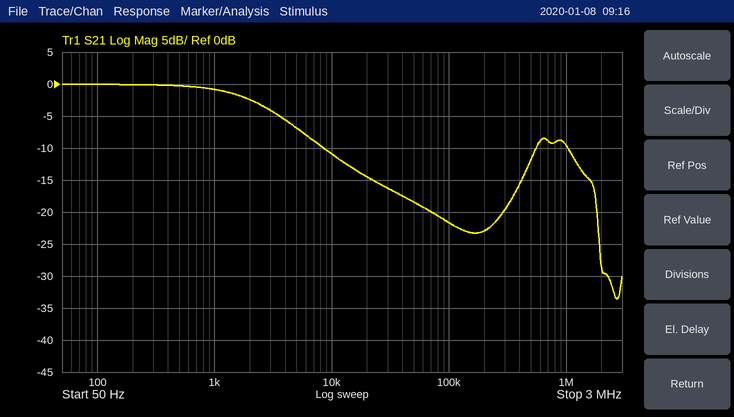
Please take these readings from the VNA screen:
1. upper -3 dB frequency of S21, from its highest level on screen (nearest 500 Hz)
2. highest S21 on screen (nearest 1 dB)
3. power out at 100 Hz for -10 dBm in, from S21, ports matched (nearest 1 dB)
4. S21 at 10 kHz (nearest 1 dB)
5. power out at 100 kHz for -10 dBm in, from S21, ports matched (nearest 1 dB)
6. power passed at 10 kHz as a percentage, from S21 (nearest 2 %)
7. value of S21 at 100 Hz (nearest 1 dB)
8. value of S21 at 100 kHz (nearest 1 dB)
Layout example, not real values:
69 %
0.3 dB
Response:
2.5 kHz
0 dB
-10 dBm
-11 dB
-32 dBm
8 %
0 dB
-22 dB
